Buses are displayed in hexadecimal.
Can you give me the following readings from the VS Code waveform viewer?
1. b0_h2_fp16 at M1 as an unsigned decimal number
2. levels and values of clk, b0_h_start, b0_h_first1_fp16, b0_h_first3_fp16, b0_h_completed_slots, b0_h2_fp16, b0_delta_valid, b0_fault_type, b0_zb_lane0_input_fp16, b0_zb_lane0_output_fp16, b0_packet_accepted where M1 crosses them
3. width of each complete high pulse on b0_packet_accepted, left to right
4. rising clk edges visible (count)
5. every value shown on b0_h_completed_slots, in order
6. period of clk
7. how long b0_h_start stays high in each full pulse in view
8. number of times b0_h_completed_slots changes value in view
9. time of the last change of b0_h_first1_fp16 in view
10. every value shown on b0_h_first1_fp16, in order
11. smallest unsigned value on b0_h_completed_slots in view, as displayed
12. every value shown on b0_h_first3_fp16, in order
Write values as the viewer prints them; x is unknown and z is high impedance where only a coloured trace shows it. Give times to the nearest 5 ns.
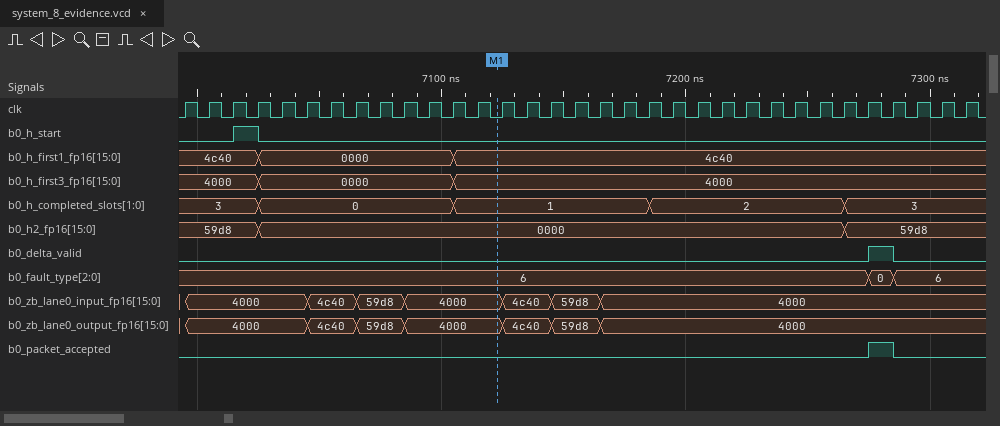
0
clk=0, b0_h_start=0, b0_h_first1_fp16=4c40, b0_h_first3_fp16=4000, b0_h_completed_slots=1, b0_h2_fp16=0000, b0_delta_valid=0, b0_fault_type=6, b0_zb_lane0_input_fp16=4000, b0_zb_lane0_output_fp16=4000, b0_packet_accepted=0
10 ns
33
3, 0, 1, 2, 3
10 ns
10 ns
4
7105 ns
4c40, 0000, 4c40
0
4000, 0000, 4000
